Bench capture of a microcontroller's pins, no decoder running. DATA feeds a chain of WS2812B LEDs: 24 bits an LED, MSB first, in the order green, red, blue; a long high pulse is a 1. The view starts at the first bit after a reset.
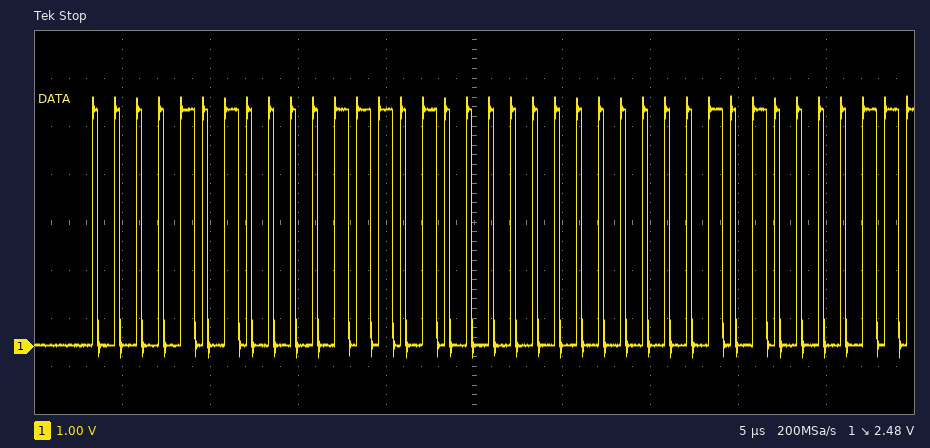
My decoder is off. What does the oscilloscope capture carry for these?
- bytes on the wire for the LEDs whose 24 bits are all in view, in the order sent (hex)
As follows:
0A 1D 00
